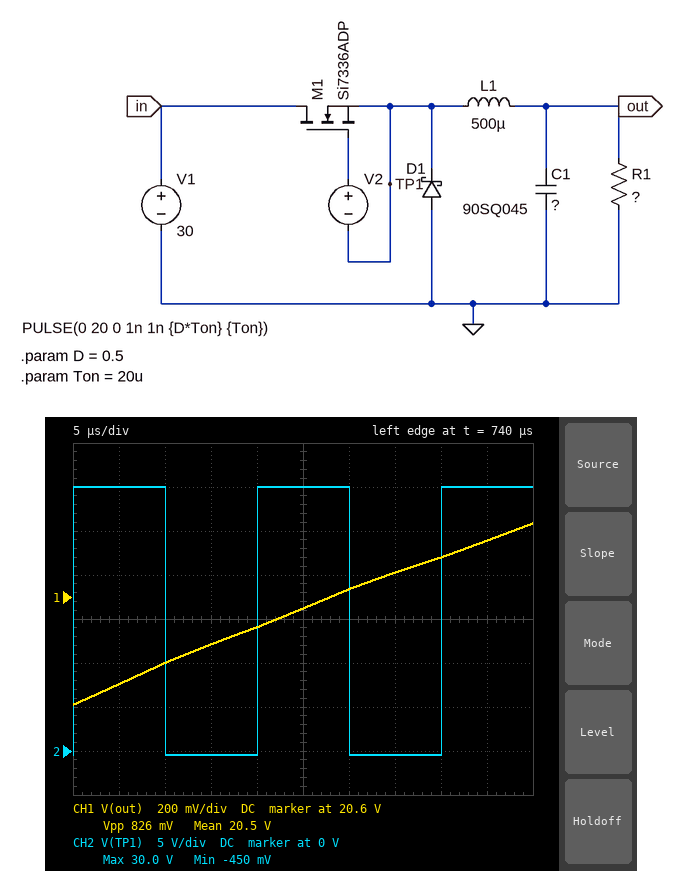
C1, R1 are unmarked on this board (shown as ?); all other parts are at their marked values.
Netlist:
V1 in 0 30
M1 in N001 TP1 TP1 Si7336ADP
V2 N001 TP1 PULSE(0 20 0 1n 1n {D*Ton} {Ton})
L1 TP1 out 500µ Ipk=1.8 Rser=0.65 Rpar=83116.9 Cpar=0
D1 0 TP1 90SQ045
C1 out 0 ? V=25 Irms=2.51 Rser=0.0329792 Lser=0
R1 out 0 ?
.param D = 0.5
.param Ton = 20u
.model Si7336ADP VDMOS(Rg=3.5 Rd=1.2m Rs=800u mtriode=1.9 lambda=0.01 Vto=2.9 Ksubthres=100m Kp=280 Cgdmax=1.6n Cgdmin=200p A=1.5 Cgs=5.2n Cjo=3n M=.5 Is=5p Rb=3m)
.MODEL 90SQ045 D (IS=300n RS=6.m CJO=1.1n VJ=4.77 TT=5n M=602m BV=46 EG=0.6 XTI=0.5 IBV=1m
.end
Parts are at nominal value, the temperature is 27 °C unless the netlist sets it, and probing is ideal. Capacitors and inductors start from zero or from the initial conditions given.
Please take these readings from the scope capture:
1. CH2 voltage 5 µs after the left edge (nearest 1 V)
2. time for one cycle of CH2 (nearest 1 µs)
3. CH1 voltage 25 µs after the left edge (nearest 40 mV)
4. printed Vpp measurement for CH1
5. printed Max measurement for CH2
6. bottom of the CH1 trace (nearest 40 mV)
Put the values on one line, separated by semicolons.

30 V; 20 µs; 20.56 V; 826 mV; 30.0 V; 20.12 V
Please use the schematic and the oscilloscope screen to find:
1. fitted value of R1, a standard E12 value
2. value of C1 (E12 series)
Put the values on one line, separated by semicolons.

68 Ω; 180 µF
